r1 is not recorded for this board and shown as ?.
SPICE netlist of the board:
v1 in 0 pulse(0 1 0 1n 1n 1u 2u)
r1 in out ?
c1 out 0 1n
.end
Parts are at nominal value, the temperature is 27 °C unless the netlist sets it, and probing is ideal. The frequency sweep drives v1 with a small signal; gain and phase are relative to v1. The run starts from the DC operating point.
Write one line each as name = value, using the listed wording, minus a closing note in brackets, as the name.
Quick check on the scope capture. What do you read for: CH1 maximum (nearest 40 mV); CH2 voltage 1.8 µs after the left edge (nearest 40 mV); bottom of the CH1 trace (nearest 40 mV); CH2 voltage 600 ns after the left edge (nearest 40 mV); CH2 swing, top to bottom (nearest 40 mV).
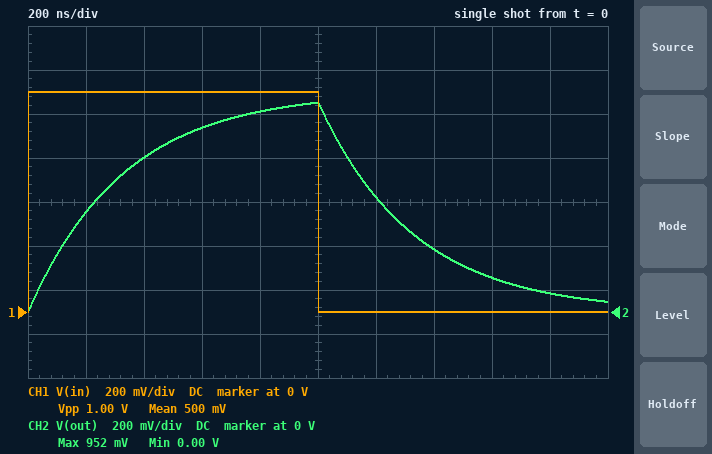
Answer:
CH1 maximum = 1.00 V
CH2 voltage 1.8 µs after the left edge = 80 mV
bottom of the CH1 trace = 0 V
CH2 voltage 600 ns after the left edge = 840 mV
CH2 swing, top to bottom = 960 mV
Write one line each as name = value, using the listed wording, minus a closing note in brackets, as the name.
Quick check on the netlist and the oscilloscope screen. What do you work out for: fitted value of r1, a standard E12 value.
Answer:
fitted value of r1, a standard E12 value = 330 Ω
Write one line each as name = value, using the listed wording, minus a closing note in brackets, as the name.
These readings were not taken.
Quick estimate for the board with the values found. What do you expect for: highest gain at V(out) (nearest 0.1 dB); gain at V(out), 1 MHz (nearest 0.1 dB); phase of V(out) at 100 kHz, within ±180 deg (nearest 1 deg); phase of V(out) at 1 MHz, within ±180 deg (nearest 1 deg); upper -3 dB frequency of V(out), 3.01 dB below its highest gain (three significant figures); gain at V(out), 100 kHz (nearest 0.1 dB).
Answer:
highest gain at V(out) = 0 dB
gain at V(out), 1 MHz = -7.2 dB
phase of V(out) at 100 kHz, within ±180 deg = -12 deg
phase of V(out) at 1 MHz, within ±180 deg = -64 deg
upper -3 dB frequency of V(out), 3.01 dB below its highest gain = 482 kHz
gain at V(out), 100 kHz = -0.2 dB
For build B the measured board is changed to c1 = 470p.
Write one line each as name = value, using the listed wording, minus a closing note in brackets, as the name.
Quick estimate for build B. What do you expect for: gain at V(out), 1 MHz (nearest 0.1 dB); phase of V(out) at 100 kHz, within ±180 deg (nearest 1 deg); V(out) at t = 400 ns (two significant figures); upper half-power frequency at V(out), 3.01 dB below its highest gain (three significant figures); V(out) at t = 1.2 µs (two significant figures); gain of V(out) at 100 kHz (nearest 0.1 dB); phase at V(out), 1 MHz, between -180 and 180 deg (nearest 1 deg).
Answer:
gain at V(out), 1 MHz = -2.9 dB
phase of V(out) at 100 kHz, within ±180 deg = -6 deg
V(out) at t = 400 ns = 920 mV
upper half-power frequency at V(out), 3.01 dB below its highest gain = 1.03 MHz
V(out) at t = 1.2 µs = 280 mV
gain of V(out) at 100 kHz = 0 dB
phase at V(out), 1 MHz, between -180 and 180 deg = -44 deg
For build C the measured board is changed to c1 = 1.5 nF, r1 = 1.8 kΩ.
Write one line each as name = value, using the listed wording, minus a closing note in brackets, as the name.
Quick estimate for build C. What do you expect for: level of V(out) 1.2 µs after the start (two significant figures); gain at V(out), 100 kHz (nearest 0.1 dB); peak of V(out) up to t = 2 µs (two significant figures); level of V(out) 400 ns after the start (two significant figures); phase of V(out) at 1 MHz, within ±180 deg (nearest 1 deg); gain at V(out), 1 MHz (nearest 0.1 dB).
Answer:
level of V(out) 1.2 µs after the start = 290 mV
gain at V(out), 100 kHz = -5.9 dB
peak of V(out) up to t = 2 µs = 310 mV
level of V(out) 400 ns after the start = 140 mV
phase of V(out) at 1 MHz, within ±180 deg = -87 deg
gain at V(out), 1 MHz = -24.6 dB
